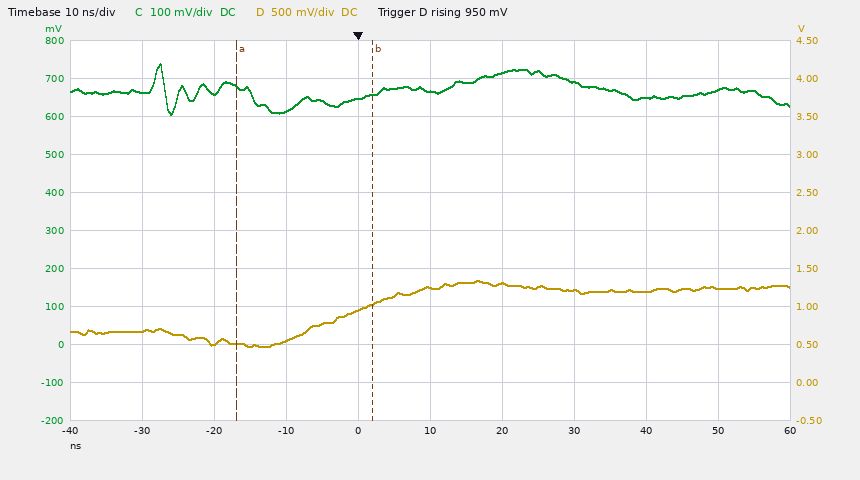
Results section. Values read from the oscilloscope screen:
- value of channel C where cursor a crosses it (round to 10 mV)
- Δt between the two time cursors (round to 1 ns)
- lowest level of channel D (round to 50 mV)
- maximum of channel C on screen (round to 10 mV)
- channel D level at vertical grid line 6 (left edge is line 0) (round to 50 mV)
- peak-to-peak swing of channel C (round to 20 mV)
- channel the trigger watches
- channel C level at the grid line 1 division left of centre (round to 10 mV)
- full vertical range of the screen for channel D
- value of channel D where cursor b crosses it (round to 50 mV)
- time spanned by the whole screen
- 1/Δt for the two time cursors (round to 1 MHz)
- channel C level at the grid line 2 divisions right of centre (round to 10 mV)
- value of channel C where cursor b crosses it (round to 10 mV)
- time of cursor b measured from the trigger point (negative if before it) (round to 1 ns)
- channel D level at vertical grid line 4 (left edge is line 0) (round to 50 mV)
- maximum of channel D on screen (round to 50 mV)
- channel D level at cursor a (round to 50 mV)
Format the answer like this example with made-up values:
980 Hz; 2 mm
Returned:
680 mV; 19 ns; 450 mV; 740 mV; 1.30 V; 140 mV; channel D; 650 mV; 5 V; 1.05 V; 100 ns; 53 MHz; 690 mV; 660 mV; +2 ns; 950 mV; 1.35 V; 500 mV
